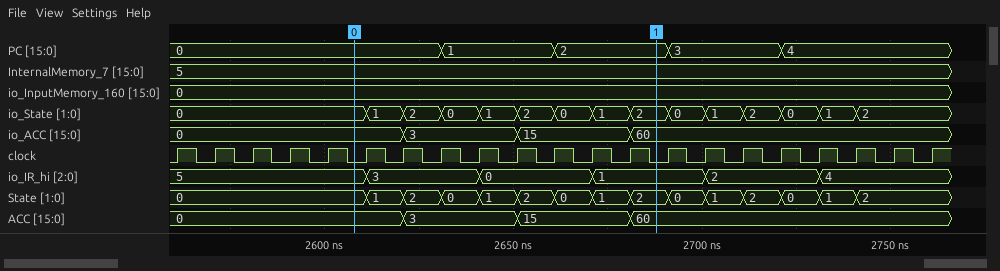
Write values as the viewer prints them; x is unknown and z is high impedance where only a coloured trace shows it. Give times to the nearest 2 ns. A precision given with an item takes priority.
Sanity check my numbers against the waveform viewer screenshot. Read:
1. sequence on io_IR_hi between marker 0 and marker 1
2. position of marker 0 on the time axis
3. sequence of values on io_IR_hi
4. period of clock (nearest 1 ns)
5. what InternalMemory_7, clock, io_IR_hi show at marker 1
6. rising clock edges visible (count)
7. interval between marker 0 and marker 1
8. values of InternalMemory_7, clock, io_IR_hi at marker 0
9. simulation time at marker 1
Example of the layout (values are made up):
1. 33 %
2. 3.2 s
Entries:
1. 5, 3, 0, 1
2. 2608 ns
3. 5, 3, 0, 1, 2, 4
4. 10 ns
5. InternalMemory_7=5, clock=0, io_IR_hi=1
6. 21
7. 80 ns
8. InternalMemory_7=5, clock=0, io_IR_hi=5
9. 2688 ns
